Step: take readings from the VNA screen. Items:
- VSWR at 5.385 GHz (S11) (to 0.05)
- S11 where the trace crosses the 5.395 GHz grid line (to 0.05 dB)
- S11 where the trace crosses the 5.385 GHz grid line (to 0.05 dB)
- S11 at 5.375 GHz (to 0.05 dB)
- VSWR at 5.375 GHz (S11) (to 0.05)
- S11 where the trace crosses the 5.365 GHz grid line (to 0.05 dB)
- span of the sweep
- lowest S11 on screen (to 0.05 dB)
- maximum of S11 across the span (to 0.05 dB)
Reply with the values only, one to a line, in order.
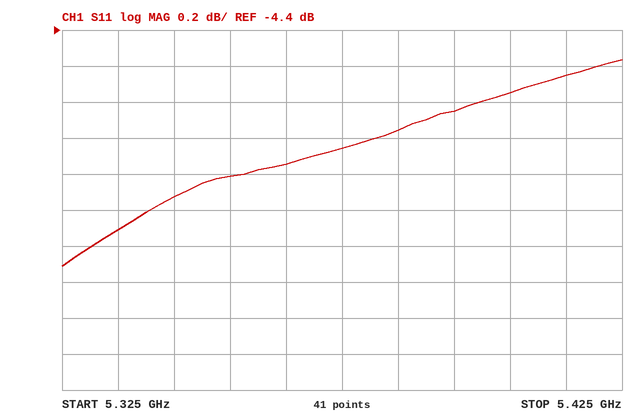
3.60
-4.85 dB
-4.95 dB
-5.05 dB
3.55
-5.15 dB
100 MHz
-5.70 dB
-4.55 dB
